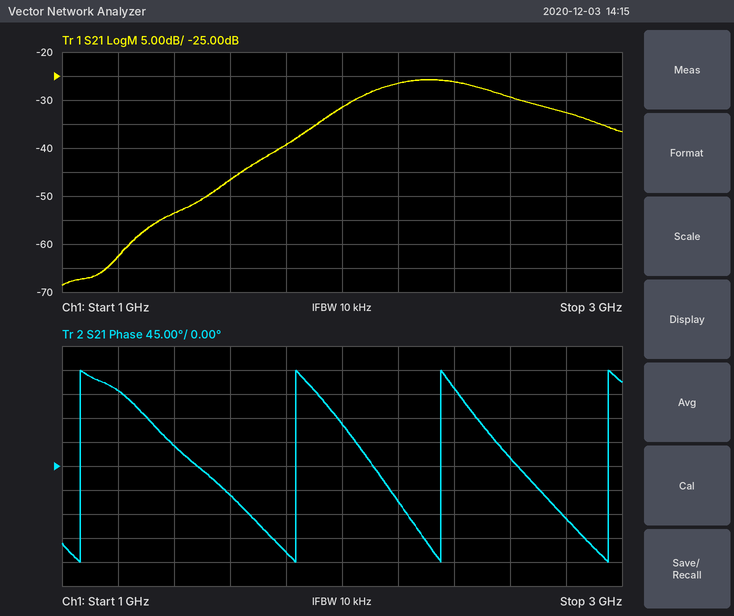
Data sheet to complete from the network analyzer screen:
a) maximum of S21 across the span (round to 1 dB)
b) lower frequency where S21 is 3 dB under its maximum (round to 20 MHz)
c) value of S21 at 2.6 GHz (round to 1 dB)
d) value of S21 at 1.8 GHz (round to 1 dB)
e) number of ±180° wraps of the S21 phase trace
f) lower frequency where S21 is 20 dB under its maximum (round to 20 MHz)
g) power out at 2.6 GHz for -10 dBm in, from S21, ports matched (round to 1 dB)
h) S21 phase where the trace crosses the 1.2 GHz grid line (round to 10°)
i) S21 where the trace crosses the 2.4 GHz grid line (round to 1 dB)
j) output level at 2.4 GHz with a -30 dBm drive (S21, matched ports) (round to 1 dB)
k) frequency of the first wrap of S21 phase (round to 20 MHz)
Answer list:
-26 dB
2.08 GHz
-29 dB
-39 dB
4
1.62 GHz
-39 dBm
140°
-26 dB
-56 dBm
1.06 GHz
